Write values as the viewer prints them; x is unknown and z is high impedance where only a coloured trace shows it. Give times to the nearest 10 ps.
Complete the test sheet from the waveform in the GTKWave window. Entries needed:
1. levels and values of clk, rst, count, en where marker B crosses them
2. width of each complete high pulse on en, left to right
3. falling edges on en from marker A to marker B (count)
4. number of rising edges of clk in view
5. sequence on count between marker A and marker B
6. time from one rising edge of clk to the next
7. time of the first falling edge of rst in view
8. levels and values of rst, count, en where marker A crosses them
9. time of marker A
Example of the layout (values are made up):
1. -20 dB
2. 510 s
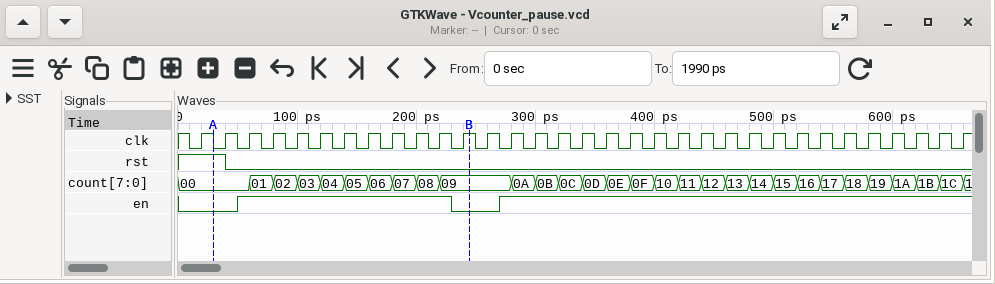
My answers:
1. clk=1, rst=0, count=09, en=0
2. 180 ps
3. 1
4. 33
5. 00, 01, 02, 03, 04, 05, 06, 07, 08, 09
6. 20 ps
7. 40 ps
8. rst=1, count=00, en=0
9. 30 ps
